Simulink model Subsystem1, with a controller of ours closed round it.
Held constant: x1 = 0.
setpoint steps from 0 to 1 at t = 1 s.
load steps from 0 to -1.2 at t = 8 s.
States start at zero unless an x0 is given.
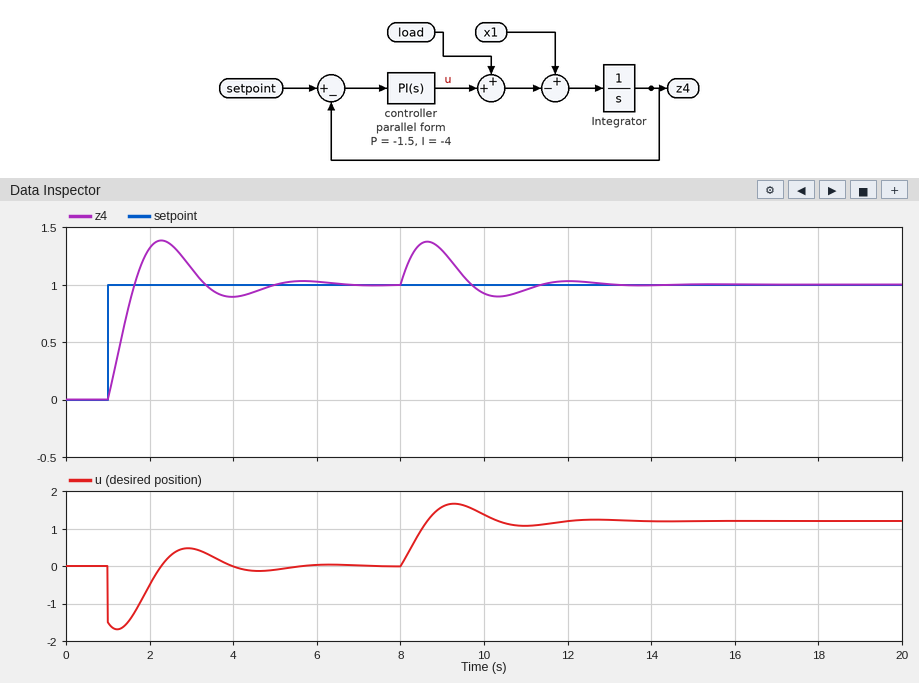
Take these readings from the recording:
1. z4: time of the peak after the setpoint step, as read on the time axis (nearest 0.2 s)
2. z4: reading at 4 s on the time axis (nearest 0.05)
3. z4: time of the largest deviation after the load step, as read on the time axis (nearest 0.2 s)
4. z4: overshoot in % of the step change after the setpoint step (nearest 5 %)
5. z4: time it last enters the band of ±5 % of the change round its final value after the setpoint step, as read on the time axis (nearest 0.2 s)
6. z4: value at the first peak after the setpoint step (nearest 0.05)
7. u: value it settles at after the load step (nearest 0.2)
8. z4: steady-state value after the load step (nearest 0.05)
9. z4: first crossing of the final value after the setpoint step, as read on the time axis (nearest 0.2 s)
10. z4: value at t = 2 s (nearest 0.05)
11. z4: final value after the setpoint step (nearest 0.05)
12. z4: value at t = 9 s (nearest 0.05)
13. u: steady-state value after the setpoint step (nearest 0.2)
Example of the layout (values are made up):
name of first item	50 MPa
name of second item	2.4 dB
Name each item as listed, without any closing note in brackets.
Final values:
z4: time of the peak after the setpoint step, as read on the time axis	2.2 s
z4: reading at 4 s on the time axis	0.90
z4: time of the largest deviation after the load step, as read on the time axis	8.6 s
z4: overshoot in % of the step change after the setpoint step	40 %
z4: time it last enters the band of ±5 % of the change round its final value after the setpoint step, as read on the time axis	4.6 s
z4: value at the first peak after the setpoint step	1.40
u: value it settles at after the load step	1.2
z4: steady-state value after the load step	1.00
z4: first crossing of the final value after the setpoint step, as read on the time axis	1.6 s
z4: value at t = 2 s	1.30
z4: final value after the setpoint step	1.00
z4: value at t = 9 s	1.30
u: steady-state value after the setpoint step	0.0
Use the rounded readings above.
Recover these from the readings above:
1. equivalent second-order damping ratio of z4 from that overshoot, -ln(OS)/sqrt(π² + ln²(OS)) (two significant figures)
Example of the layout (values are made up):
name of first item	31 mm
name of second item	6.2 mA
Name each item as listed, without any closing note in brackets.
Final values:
equivalent second-order damping ratio of z4 from that overshoot, -ln(OS)/sqrt(π² + ln²(OS))	0.28
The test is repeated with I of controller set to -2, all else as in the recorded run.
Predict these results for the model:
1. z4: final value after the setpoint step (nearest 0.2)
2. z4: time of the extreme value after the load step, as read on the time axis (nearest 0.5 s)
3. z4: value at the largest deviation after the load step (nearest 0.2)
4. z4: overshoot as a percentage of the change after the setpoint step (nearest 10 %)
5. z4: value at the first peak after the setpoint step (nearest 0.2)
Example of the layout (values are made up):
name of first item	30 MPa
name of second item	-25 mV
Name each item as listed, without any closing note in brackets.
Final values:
z4: final value after the setpoint step	1.0
z4: time of the extreme value after the load step, as read on the time axis	9.0 s
z4: value at the largest deviation after the load step	1.4
z4: overshoot as a percentage of the change after the setpoint step	30 %
z4: value at the first peak after the setpoint step	1.2
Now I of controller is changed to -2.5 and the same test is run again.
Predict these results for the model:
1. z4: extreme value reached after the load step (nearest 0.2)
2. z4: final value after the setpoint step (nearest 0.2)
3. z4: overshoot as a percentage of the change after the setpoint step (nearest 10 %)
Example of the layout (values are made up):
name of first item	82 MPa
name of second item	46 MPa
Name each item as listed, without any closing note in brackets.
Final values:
z4: extreme value reached after the load step	1.4
z4: final value after the setpoint step	1.0
z4: overshoot as a percentage of the change after the setpoint step	30 %
